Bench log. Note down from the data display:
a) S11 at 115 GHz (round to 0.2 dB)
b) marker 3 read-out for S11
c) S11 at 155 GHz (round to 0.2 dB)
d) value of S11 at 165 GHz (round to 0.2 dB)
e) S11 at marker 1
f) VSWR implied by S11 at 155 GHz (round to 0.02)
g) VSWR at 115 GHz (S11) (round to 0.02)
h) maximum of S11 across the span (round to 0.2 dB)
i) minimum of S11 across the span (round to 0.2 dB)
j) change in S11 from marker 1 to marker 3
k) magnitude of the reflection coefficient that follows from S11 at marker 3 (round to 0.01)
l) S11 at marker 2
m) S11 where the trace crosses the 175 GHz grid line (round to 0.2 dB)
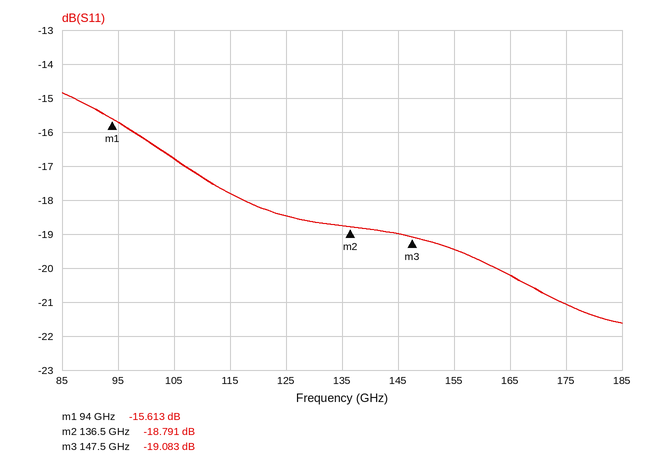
-17.8 dB
-19.083 dB
-19.4 dB
-20.2 dB
-15.613 dB
1.24
1.30
-14.8 dB
-21.6 dB
-3.470 dB
0.11
-18.791 dB
-21.0 dB
